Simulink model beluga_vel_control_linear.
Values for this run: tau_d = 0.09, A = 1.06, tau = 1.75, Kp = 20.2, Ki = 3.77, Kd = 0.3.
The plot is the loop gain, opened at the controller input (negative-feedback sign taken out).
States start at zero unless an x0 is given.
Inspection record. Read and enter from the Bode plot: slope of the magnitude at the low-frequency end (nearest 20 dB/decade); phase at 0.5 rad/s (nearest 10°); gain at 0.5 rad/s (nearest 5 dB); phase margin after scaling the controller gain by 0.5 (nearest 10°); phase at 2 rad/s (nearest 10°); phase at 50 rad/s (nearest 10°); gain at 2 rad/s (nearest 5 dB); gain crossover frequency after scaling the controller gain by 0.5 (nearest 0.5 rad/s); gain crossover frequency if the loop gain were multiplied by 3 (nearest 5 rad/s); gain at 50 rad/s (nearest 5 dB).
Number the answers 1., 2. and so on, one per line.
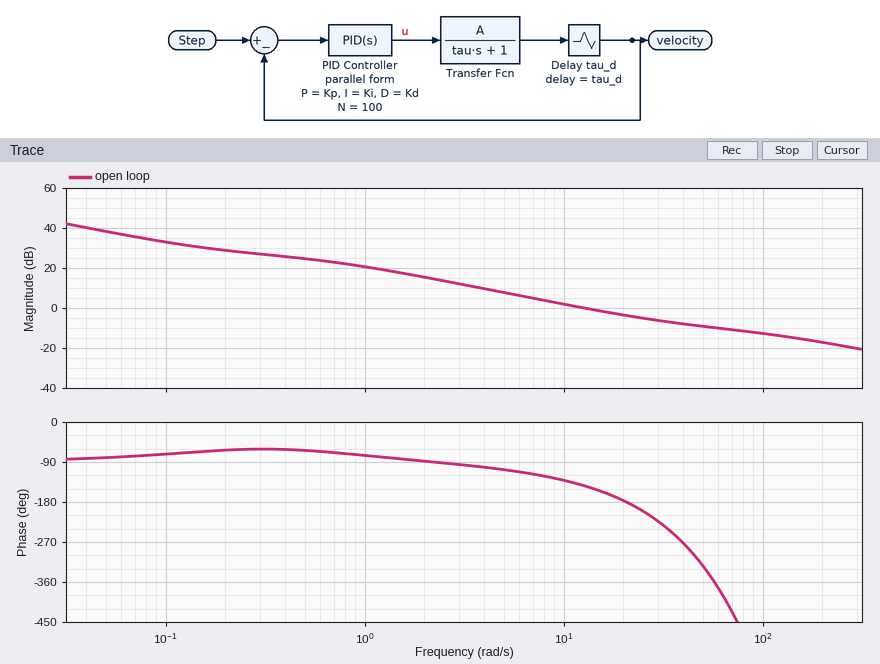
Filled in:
1. -20 dB/decade
2. -60°
3. 25 dB
4. 70°
5. -90°
6. -320°
7. 15 dB
8. 6.0 rad/s
9. 55 rad/s
10. -10 dB
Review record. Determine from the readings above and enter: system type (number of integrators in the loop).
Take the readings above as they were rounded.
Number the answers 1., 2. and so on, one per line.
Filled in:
1. 1
